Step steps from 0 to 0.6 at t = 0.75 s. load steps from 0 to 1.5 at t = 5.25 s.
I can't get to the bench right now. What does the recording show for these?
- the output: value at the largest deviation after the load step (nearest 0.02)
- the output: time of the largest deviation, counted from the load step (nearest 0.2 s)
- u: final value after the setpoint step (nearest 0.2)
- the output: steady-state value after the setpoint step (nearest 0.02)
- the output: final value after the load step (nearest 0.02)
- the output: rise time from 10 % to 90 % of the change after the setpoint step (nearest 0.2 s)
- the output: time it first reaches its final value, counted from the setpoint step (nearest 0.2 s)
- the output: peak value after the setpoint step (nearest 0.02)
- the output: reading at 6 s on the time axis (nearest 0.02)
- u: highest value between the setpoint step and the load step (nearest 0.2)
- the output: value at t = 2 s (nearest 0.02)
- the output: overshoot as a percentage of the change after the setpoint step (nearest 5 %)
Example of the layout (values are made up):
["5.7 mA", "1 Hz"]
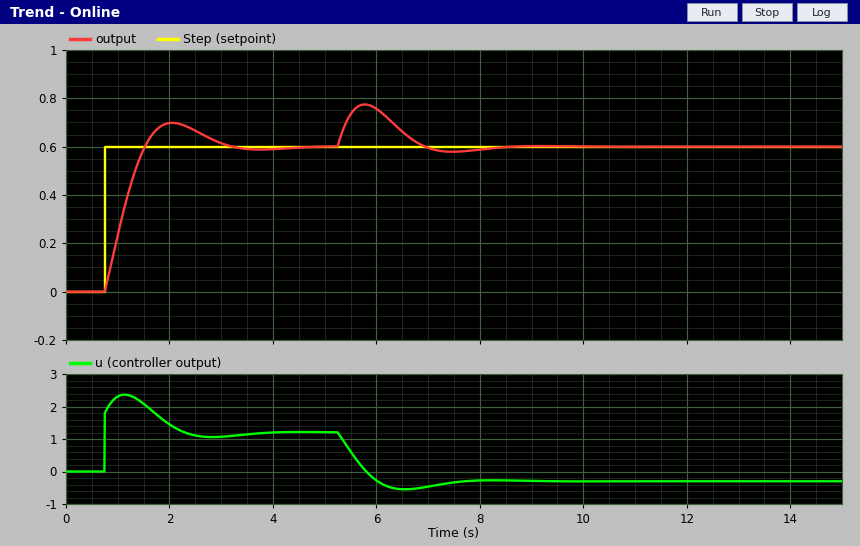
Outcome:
["0.78", "0.6 s", "1.2", "0.60", "0.60", "0.6 s", "0.8 s", "0.70", "0.76", "2.4", "0.70", "15 %"]
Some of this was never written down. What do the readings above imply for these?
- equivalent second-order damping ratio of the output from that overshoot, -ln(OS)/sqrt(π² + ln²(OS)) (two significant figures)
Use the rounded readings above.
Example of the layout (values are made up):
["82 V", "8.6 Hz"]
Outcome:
["0.52"]
